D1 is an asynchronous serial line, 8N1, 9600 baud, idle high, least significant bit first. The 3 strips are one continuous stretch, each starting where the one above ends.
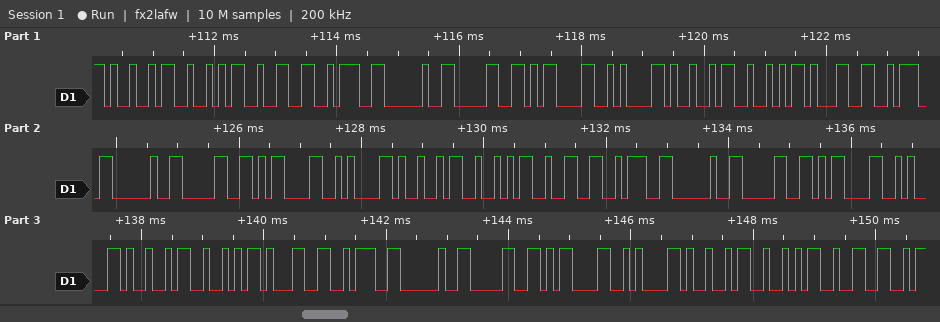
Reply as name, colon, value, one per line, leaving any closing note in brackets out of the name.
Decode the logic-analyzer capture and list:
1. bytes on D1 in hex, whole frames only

bytes on D1 in hex, whole frames only: 49 52 32 3A 20 30 0D 0A 49 52 31 3A 20 30 0D 0A 49 52 32 3A 20 30 0D 0A 49 52 31 3A 20 30 0D 0A 49 52 32
